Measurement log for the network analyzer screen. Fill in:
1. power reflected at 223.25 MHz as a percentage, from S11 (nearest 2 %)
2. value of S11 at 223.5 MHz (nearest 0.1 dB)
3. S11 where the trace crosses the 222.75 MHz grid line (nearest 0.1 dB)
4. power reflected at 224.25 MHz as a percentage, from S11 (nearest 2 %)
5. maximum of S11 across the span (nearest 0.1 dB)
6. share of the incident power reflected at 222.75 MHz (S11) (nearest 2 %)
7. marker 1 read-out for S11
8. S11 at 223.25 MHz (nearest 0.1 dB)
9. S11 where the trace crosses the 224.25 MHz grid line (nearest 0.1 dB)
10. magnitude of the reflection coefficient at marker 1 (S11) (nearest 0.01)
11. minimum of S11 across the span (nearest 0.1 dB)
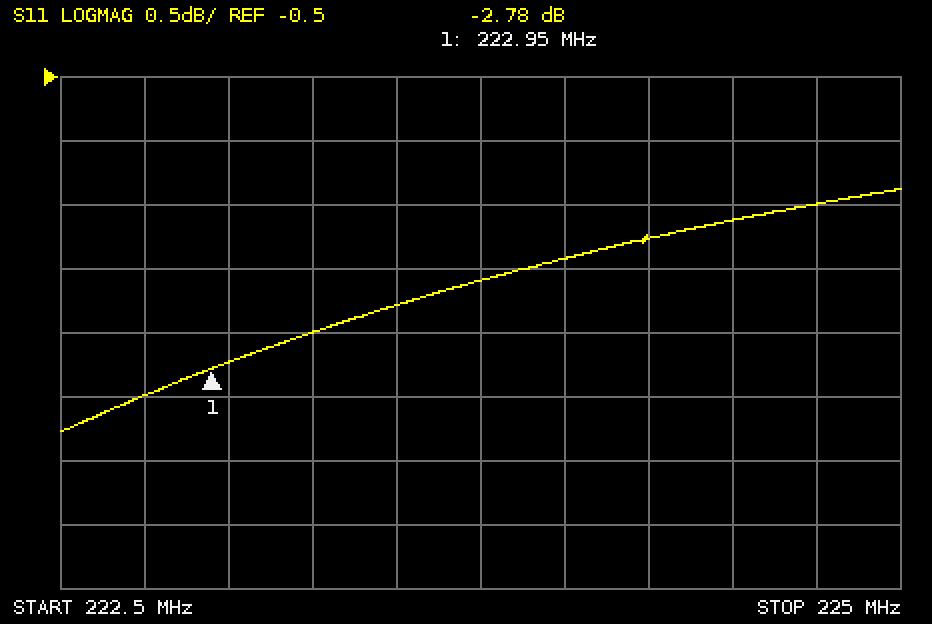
56 %
-2.3 dB
-3.0 dB
66 %
-1.4 dB
50 %
-2.78 dB
-2.5 dB
-1.8 dB
0.73
-3.3 dB
